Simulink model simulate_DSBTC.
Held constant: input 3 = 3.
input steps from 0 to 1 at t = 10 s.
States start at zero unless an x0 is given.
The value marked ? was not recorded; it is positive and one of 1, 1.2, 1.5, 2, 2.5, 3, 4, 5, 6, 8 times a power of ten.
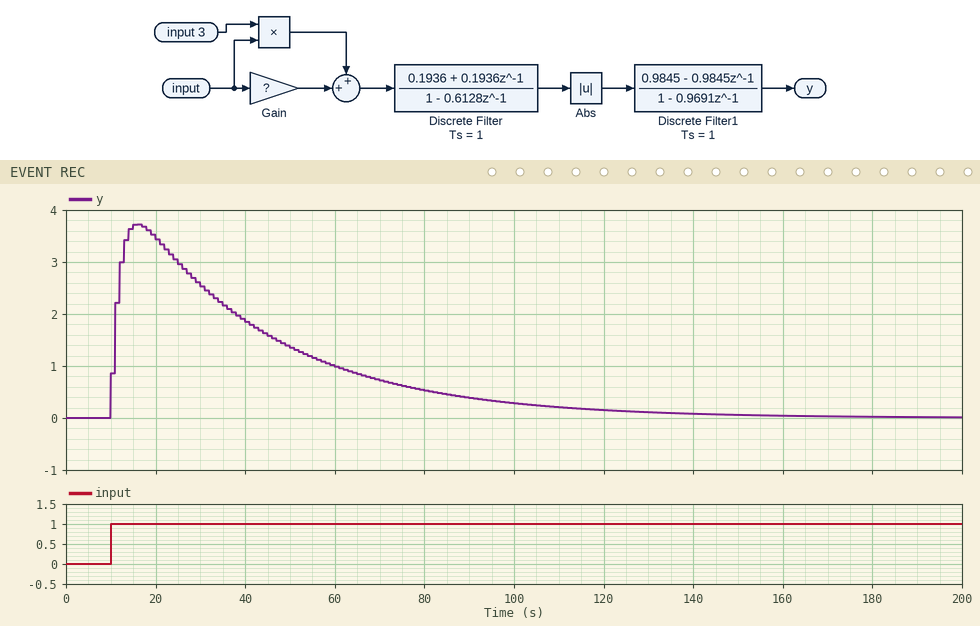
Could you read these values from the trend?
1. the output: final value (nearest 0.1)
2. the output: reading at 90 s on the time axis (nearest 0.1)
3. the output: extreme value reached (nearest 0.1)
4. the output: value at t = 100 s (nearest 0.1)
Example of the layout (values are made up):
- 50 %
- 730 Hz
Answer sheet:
- 0.0
- 0.4
- 3.7
- 0.3
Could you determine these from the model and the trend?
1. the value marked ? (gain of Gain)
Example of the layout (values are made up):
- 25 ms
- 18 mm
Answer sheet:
- 1.5
